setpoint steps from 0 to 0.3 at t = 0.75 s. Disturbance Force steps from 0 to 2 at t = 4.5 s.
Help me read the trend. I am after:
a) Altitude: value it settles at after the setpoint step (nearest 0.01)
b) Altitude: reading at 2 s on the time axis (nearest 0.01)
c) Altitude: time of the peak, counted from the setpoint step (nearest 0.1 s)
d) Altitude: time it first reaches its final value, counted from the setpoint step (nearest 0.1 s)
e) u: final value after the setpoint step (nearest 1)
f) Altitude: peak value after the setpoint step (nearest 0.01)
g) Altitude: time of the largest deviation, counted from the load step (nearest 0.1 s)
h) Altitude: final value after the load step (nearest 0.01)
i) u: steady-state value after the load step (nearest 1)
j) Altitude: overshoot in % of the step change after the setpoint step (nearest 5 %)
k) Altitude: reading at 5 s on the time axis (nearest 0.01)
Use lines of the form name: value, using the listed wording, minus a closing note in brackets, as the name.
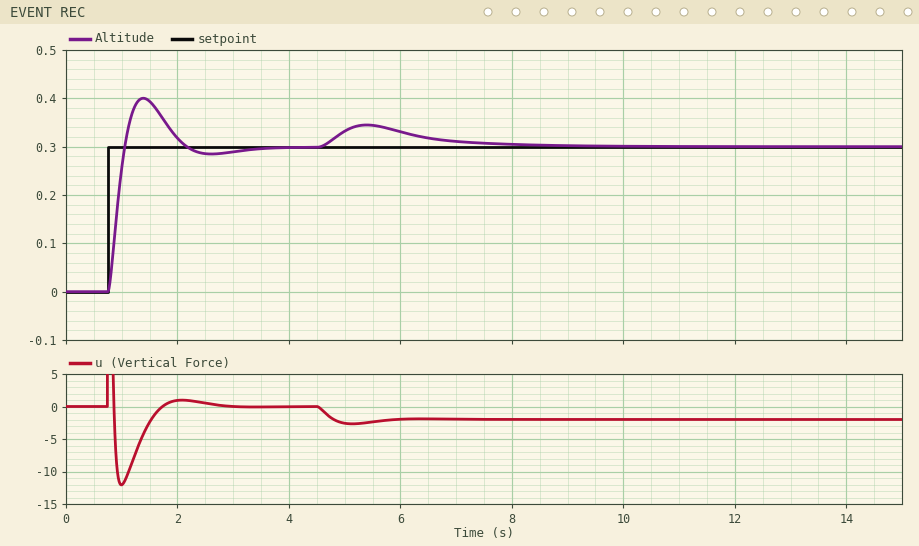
Altitude: value it settles at after the setpoint step: 0.30
Altitude: reading at 2 s on the time axis: 0.32
Altitude: time of the peak, counted from the setpoint step: 0.6 s
Altitude: time it first reaches its final value, counted from the setpoint step: 0.3 s
u: final value after the setpoint step: 0
Altitude: peak value after the setpoint step: 0.40
Altitude: time of the largest deviation, counted from the load step: 0.9 s
Altitude: final value after the load step: 0.30
u: steady-state value after the load step: -2
Altitude: overshoot in % of the step change after the setpoint step: 35 %
Altitude: reading at 5 s on the time axis: 0.33
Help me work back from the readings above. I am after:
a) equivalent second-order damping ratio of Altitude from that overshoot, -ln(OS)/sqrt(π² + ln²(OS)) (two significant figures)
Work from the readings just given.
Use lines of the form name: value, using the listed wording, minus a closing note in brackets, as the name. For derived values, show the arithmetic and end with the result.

equivalent second-order damping ratio of Altitude from that overshoot, -ln(OS)/sqrt(π² + ln²(OS)): ln(0.35) = -1.050; 1.050 / sqrt(9.870 + 1.102) = 0.32
